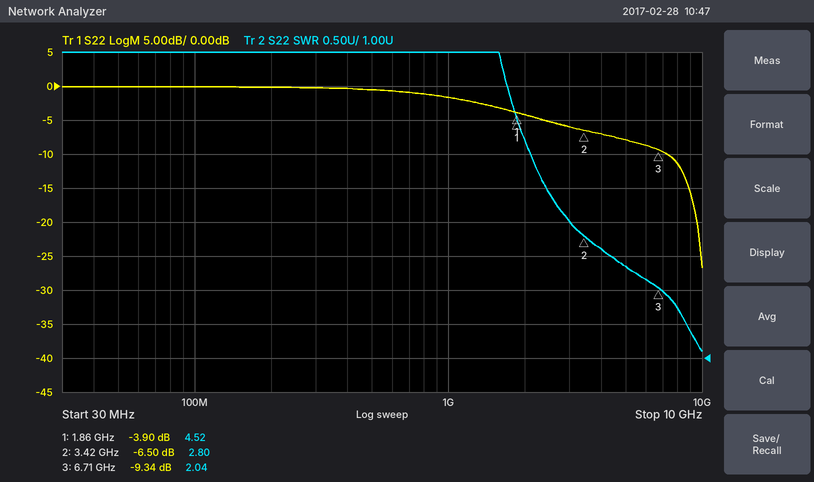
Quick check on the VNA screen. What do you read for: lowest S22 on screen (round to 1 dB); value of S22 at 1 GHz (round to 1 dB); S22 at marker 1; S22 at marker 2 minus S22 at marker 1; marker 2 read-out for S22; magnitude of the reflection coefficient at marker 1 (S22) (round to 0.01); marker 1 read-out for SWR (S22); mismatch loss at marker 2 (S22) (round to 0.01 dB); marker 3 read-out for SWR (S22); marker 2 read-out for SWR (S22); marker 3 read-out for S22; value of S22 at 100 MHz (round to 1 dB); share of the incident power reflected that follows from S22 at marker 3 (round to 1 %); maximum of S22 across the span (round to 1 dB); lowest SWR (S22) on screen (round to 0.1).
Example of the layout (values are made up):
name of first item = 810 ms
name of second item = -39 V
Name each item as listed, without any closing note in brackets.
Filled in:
lowest S22 on screen = -27 dB
value of S22 at 1 GHz = -2 dB
S22 at marker 1 = -3.90 dB
S22 at marker 2 minus S22 at marker 1 = -2.60 dB
marker 2 read-out for S22 = -6.50 dB
magnitude of the reflection coefficient at marker 1 (S22) = 0.64
marker 1 read-out for SWR = 4.52
mismatch loss at marker 2 (S22) = 1.10 dB
marker 3 read-out for SWR = 2.04
marker 2 read-out for SWR = 2.80
marker 3 read-out for S22 = -9.34 dB
value of S22 at 100 MHz = 0 dB
share of the incident power reflected that follows from S22 at marker 3 = 12 %
maximum of S22 across the span = 0 dB
lowest SWR (S22) on screen = 1.1
